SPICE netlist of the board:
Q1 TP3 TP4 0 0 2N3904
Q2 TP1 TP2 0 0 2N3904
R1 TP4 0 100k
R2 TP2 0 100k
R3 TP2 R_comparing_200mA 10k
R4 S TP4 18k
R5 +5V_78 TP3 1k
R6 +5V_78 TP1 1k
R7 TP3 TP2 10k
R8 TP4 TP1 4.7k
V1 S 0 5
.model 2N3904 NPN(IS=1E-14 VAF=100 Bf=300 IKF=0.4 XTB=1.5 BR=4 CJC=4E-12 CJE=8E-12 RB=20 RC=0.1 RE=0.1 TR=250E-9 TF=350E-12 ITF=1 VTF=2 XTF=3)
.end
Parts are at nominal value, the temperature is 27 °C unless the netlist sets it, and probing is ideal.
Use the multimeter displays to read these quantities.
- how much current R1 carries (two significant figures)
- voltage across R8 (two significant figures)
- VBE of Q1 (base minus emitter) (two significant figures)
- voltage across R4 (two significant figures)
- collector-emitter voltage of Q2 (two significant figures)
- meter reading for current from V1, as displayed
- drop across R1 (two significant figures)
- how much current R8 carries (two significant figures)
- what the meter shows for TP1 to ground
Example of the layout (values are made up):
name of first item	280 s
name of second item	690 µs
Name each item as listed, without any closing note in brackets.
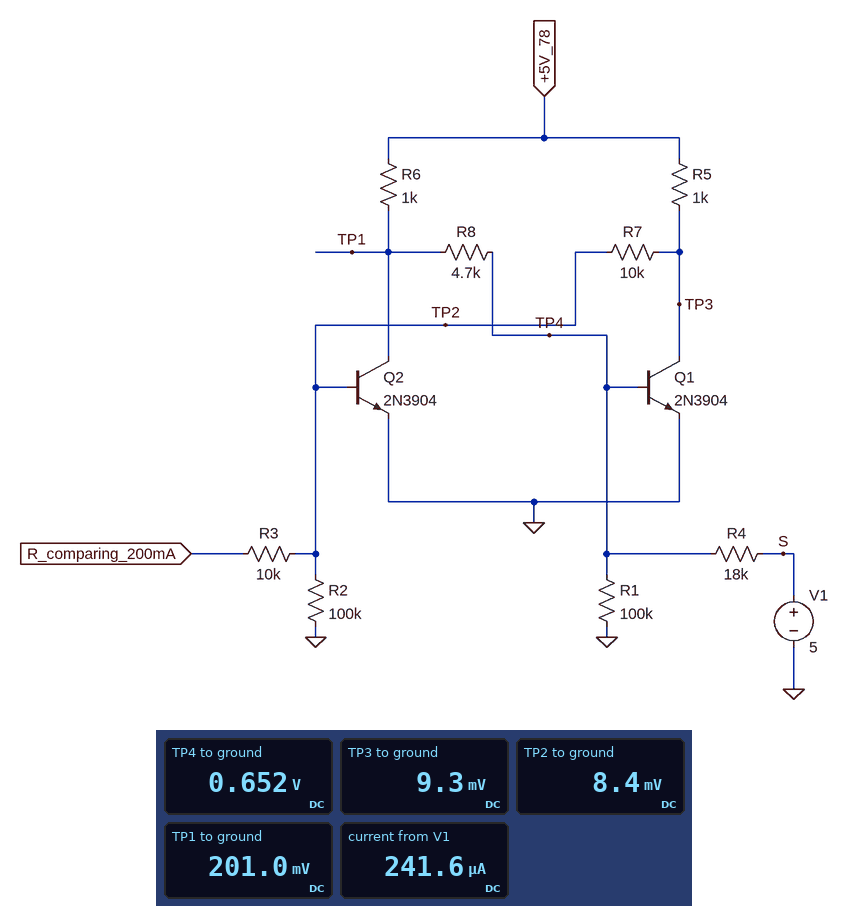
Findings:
how much current R1 carries	6.5 µA
voltage across R8	450 mV
VBE of Q1 (base minus emitter)	650 mV
voltage across R4	4.3 V
collector-emitter voltage of Q2	200 mV
meter reading for current from V1, as displayed	241.6 µA
drop across R1	650 mV
how much current R8 carries	96 µA
what the meter shows for TP1 to ground	201.0 mV
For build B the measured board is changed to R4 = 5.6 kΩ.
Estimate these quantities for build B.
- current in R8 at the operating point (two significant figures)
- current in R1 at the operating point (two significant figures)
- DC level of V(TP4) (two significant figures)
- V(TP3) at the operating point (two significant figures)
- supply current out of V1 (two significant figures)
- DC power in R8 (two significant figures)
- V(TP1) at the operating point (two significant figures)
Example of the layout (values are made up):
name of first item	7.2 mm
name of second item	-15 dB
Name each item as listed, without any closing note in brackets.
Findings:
current in R8 at the operating point	100 µA
current in R1 at the operating point	7.0 µA
DC level of V(TP4)	700 mV
V(TP3) at the operating point	6.8 mV
supply current out of V1	770 µA
DC power in R8	50 µW
V(TP1) at the operating point	210 mV
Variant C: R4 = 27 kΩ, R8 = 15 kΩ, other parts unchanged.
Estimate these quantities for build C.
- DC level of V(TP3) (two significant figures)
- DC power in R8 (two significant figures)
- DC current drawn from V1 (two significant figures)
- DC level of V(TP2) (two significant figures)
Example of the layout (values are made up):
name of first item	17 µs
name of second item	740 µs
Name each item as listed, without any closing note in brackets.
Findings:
DC level of V(TP3)	7.5 mV
DC power in R8	21 µW
DC current drawn from V1	160 µA
DC level of V(TP2)	6.8 mV
